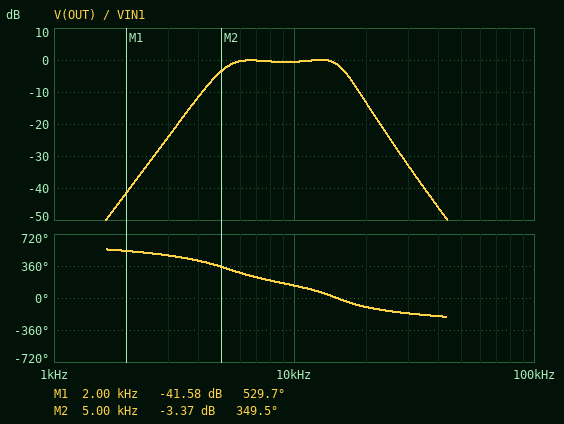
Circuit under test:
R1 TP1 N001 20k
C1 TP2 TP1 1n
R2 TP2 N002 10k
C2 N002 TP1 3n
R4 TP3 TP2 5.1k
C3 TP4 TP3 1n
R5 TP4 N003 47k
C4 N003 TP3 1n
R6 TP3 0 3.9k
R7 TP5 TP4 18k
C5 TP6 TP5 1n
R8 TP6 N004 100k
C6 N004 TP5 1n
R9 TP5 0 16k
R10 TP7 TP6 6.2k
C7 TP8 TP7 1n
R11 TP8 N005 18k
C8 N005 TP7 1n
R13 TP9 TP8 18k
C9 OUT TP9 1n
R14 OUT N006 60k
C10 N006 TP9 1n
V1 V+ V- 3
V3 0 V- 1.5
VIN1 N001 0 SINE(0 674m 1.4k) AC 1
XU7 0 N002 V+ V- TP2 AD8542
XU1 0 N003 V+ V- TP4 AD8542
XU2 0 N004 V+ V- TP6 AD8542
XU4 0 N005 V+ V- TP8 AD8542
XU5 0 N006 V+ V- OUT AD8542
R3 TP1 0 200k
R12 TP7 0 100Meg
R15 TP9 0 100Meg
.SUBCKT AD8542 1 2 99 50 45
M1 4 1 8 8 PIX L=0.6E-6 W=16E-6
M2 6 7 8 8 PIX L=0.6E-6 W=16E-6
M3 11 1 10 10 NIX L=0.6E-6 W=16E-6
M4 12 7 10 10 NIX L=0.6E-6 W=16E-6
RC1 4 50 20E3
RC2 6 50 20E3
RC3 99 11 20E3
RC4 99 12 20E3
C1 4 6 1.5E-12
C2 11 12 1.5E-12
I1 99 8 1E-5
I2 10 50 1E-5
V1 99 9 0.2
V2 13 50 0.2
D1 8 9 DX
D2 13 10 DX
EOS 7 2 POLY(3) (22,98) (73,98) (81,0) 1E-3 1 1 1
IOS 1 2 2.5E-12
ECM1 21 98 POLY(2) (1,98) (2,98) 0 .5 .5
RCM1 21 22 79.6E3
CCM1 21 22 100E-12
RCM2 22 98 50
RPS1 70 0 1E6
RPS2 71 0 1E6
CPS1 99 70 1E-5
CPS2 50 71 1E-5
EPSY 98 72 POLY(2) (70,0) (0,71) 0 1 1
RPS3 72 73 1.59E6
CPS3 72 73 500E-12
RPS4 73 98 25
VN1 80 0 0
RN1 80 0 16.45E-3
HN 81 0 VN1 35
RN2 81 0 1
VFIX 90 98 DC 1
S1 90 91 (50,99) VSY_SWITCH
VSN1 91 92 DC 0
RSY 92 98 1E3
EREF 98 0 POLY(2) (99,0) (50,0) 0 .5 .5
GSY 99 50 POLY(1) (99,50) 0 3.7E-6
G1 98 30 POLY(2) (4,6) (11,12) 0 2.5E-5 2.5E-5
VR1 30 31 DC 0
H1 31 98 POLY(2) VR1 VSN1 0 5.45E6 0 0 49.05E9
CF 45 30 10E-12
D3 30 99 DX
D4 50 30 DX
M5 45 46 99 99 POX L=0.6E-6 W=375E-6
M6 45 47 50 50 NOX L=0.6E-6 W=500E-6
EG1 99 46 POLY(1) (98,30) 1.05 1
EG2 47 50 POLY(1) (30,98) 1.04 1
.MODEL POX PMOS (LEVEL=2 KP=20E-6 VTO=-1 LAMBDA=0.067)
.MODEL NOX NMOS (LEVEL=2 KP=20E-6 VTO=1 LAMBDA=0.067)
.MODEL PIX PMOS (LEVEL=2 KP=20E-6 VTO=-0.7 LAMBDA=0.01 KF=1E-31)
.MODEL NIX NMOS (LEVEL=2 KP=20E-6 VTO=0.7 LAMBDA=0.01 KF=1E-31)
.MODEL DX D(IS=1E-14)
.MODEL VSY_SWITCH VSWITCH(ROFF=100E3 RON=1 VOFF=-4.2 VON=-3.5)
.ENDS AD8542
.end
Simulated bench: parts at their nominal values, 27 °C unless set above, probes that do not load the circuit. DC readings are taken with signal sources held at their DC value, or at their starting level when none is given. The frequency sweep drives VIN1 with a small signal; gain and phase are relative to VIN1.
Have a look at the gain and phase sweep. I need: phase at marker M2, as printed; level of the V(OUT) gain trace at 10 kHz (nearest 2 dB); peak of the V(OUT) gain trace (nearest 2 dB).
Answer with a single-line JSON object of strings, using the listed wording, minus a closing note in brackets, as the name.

{"phase at marker M2, as printed": "349.5 deg", "level of the V(OUT) gain trace at 10 kHz": "0 dB", "peak of the V(OUT) gain trace": "0 dB"}
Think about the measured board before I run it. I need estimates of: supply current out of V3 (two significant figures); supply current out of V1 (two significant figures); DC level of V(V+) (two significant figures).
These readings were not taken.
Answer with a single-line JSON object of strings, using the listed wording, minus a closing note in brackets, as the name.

{"supply current out of V3": "140 nA", "supply current out of V1": "240 µA", "DC level of V(V+)": "1.5 V"}
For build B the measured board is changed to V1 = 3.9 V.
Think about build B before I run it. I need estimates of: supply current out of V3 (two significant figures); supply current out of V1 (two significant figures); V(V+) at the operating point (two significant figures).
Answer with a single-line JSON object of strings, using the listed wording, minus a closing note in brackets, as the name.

{"supply current out of V3": "100 nA", "supply current out of V1": "260 µA", "V(V+) at the operating point": "2.4 V"}
